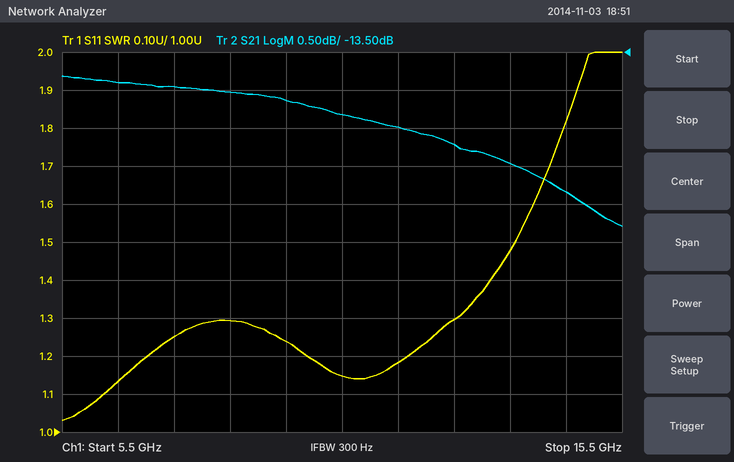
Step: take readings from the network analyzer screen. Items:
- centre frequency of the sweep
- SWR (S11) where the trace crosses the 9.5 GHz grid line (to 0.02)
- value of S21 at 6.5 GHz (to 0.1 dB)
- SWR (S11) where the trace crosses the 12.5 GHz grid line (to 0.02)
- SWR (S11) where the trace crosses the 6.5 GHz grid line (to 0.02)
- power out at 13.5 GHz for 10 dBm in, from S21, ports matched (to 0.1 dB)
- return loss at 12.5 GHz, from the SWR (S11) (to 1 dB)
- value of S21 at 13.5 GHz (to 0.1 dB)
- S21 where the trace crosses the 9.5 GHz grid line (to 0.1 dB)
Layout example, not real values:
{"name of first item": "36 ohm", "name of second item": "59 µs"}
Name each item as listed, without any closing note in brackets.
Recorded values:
{"centre frequency of the sweep": "10.5 GHz", "SWR (S11) where the trace crosses the 9.5 GHz grid line": "1.24", "value of S21 at 6.5 GHz": "-13.9 dB", "SWR (S11) where the trace crosses the 12.5 GHz grid line": "1.30", "SWR (S11) where the trace crosses the 6.5 GHz grid line": "1.14", "power out at 13.5 GHz for 10 dBm in, from S21, ports matched": "-5.0 dBm", "return loss at 12.5 GHz, from the SWR (S11)": "18 dB", "value of S21 at 13.5 GHz": "-15.0 dB", "S21 where the trace crosses the 9.5 GHz grid line": "-14.1 dB"}
